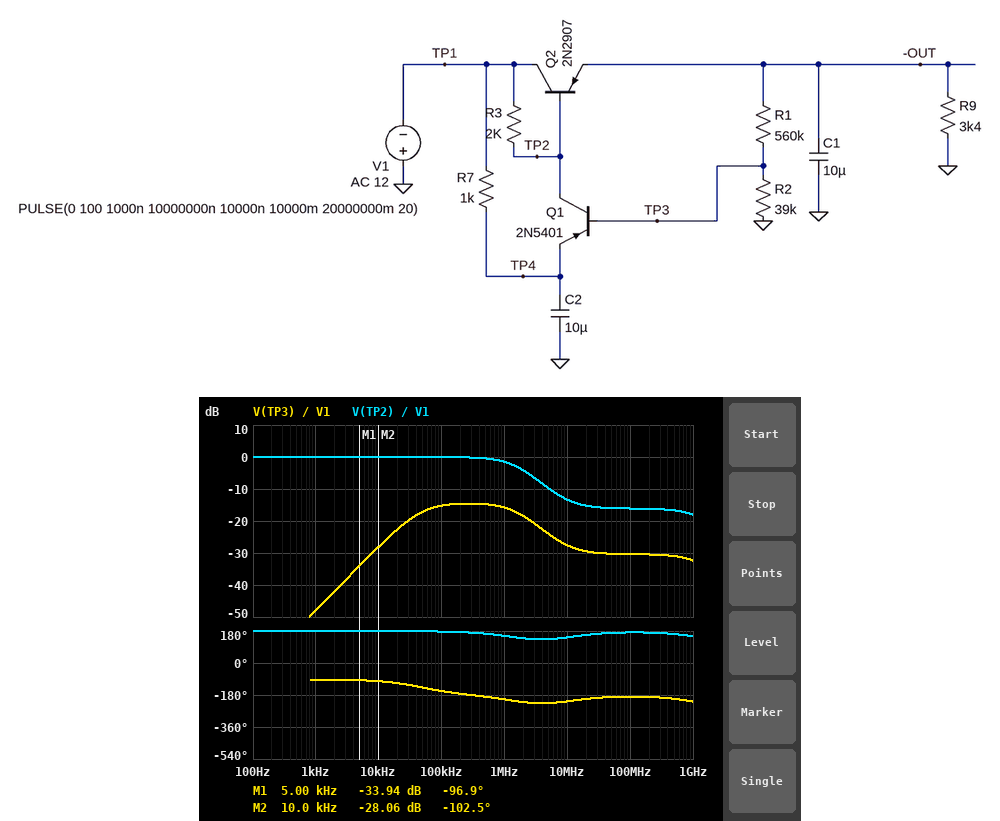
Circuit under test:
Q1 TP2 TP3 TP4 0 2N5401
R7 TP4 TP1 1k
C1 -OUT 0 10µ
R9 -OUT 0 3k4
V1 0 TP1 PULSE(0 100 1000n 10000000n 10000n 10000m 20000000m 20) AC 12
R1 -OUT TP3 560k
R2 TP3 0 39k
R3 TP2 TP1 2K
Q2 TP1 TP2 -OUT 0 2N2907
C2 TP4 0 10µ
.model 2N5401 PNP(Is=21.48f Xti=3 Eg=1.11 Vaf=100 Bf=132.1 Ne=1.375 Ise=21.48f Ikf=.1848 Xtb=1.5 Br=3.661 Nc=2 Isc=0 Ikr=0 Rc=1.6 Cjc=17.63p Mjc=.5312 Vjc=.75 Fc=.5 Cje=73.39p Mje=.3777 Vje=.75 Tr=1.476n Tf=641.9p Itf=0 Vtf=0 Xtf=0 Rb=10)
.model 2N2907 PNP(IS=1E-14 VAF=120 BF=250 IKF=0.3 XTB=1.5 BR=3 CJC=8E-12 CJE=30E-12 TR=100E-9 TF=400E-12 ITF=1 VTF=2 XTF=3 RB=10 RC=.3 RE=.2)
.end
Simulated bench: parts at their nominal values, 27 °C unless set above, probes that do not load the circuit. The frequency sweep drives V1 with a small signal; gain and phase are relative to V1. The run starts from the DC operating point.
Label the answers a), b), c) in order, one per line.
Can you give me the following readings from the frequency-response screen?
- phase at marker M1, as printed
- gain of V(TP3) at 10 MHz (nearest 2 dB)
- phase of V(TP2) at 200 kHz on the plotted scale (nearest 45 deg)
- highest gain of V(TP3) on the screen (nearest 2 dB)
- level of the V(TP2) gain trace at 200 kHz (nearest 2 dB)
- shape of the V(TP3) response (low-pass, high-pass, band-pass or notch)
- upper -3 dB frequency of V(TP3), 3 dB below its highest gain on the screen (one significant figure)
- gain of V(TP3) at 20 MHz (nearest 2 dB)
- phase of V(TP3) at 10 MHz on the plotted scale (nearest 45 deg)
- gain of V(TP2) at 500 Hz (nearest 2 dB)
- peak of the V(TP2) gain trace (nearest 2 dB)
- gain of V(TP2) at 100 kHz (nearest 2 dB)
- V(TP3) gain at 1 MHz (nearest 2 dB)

a) -96.9 deg
b) -28 dB
c) 180 deg
d) -14 dB
e) 0 dB
f) band-pass
g) 2 MHz
h) -30 dB
i) -225 deg
j) 0 dB
k) 0 dB
l) 0 dB
m) -16 dB
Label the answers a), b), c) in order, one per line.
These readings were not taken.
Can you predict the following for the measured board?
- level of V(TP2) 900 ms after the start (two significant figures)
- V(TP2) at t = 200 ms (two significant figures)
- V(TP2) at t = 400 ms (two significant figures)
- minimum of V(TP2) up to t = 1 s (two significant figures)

a) -100 V
b) -100 V
c) -100 V
d) -100 V
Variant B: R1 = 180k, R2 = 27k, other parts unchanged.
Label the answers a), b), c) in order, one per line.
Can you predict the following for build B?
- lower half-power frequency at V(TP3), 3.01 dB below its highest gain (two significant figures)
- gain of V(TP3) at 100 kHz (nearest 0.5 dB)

a) 68 kHz
b) -16.0 dB
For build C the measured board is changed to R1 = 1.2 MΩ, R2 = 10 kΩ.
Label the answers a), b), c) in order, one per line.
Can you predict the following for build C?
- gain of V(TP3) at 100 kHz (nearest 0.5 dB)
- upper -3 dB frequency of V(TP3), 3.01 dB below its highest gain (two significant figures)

a) -20.5 dB
b) 1.9 MHz
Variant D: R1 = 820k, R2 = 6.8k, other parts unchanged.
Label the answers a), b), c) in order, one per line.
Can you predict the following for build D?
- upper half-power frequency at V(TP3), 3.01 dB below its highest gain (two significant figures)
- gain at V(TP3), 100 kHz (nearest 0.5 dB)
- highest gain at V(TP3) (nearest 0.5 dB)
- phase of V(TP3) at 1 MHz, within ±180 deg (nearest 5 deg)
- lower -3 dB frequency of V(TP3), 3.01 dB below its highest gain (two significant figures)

a) 2.1 MHz
b) -23.0 dB
c) -15.5 dB
d) 165 deg
e) 200 kHz
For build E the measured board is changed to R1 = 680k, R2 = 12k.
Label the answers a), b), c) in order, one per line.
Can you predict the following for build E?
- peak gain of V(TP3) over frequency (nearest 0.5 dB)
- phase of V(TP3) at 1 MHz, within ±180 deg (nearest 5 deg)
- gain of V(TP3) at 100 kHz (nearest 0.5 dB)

a) -15.0 dB
b) 160 deg
c) -19.5 dB
